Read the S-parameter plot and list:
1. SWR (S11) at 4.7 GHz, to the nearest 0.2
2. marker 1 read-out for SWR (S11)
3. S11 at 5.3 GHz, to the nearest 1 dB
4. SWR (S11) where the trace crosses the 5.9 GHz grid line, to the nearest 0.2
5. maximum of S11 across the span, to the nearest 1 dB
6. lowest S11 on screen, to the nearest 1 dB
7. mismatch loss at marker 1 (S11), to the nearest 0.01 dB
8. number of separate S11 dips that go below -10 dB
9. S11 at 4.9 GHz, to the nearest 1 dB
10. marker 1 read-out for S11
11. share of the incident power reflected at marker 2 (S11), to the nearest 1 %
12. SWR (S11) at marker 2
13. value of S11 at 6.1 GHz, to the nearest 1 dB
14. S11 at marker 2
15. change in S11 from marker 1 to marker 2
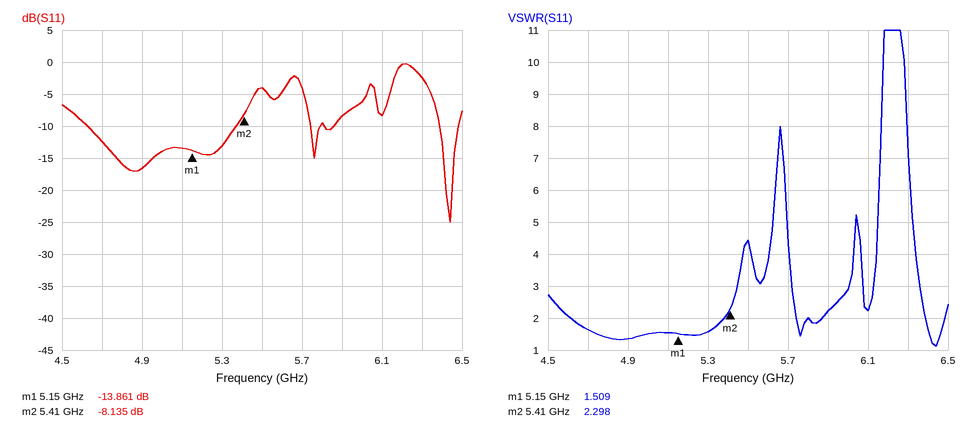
1.6
1.509
-13 dB
2.2
0 dB
-25 dB
0.18 dB
3
-17 dB
-13.861 dB
15 %
2.298
-8 dB
-8.135 dB
5.726 dB
